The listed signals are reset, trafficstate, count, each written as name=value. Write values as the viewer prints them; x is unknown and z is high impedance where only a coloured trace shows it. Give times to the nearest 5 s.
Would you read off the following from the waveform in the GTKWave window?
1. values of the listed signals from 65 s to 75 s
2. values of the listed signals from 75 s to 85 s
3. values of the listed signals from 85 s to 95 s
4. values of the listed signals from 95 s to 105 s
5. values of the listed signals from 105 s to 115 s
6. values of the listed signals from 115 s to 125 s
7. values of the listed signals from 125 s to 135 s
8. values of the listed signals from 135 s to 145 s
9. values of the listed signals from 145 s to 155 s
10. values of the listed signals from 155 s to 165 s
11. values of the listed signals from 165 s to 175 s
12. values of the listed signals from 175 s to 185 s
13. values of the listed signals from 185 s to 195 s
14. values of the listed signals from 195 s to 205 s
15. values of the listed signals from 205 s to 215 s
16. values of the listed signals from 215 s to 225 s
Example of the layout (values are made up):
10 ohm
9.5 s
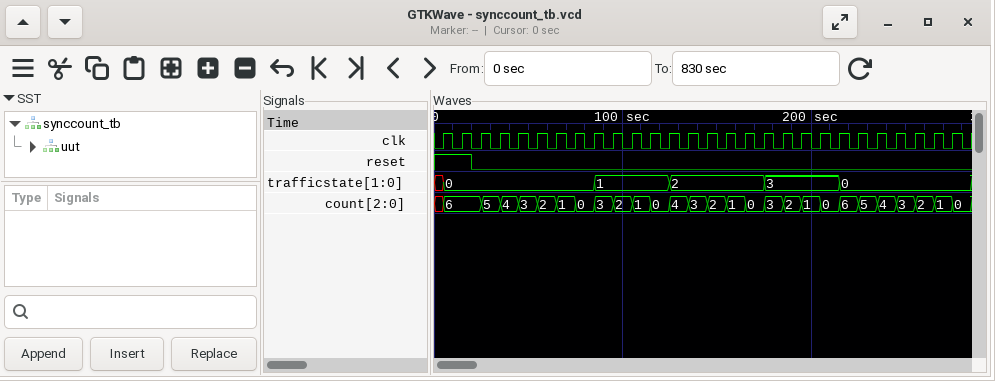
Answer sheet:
reset=0, trafficstate=0, count=1
reset=0, trafficstate=0, count=0
reset=0, trafficstate=1, count=3
reset=0, trafficstate=1, count=2
reset=0, trafficstate=1, count=1
reset=0, trafficstate=1, count=0
reset=0, trafficstate=2, count=4
reset=0, trafficstate=2, count=3
reset=0, trafficstate=2, count=2
reset=0, trafficstate=2, count=1
reset=0, trafficstate=2, count=0
reset=0, trafficstate=3, count=3
reset=0, trafficstate=3, count=2
reset=0, trafficstate=3, count=1
reset=0, trafficstate=3, count=0
reset=0, trafficstate=0, count=6
